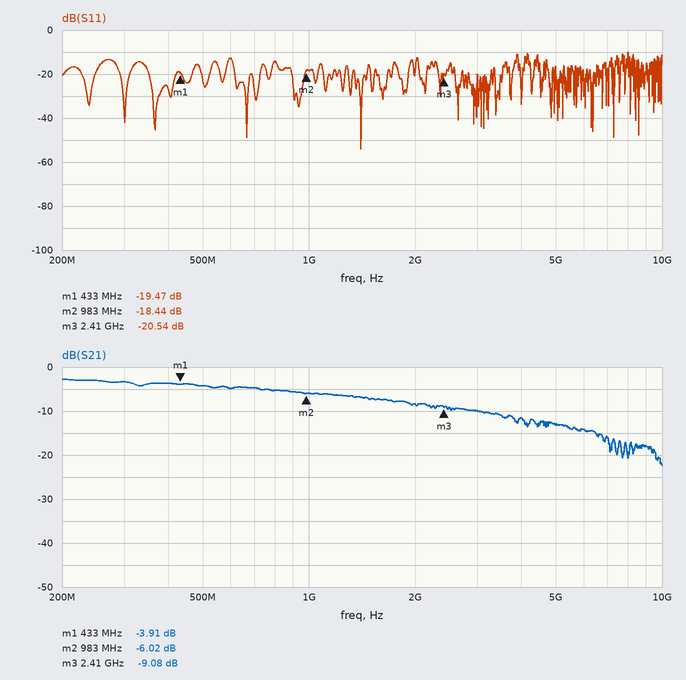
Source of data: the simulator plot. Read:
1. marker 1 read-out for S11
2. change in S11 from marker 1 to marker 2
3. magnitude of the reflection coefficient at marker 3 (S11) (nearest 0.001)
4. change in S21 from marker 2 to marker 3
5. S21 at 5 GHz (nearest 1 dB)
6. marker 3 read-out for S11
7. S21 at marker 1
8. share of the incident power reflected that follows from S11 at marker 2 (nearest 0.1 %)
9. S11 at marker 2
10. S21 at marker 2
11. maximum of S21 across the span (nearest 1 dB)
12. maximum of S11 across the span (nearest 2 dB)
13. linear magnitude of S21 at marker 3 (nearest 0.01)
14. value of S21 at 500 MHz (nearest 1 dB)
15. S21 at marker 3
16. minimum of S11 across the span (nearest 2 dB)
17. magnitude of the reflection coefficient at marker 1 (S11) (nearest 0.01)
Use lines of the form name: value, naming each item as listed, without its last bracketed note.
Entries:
marker 1 read-out for S11: -19.47 dB
change in S11 from marker 1 to marker 2: 1.03 dB
magnitude of the reflection coefficient at marker 3 (S11): 0.094
change in S21 from marker 2 to marker 3: -3.06 dB
S21 at 5 GHz: -13 dB
marker 3 read-out for S11: -20.54 dB
S21 at marker 1: -3.91 dB
share of the incident power reflected that follows from S11 at marker 2: 1.4 %
S11 at marker 2: -18.44 dB
S21 at marker 2: -6.02 dB
maximum of S21 across the span: -3 dB
maximum of S11 across the span: -10 dB
linear magnitude of S21 at marker 3: 0.35
value of S21 at 500 MHz: -4 dB
S21 at marker 3: -9.08 dB
minimum of S11 across the span: -54 dB
magnitude of the reflection coefficient at marker 1 (S11): 0.11
